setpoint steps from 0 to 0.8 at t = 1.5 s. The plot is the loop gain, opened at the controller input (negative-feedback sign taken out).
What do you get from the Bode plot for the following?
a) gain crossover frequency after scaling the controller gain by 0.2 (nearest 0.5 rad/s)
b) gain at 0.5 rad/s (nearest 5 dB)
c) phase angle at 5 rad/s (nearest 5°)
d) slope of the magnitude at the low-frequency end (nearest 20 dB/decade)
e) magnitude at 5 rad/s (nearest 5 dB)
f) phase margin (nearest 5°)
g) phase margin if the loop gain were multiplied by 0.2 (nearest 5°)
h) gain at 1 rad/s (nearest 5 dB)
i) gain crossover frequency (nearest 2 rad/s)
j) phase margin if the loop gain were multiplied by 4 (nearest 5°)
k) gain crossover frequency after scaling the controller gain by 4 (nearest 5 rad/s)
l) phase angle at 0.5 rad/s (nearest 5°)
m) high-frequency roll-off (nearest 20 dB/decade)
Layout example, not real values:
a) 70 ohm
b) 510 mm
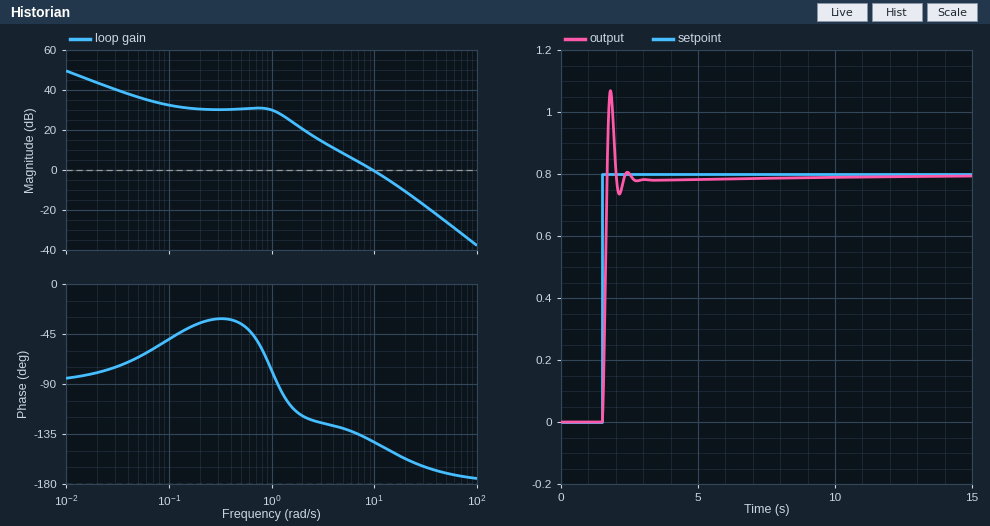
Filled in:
a) 3.0 rad/s
b) 30 dB
c) -130°
d) -20 dB/decade
e) 10 dB
f) 40°
g) 55°
h) 30 dB
i) 10 rad/s
j) 20°
k) 20 rad/s
l) -35°
m) -40 dB/decade
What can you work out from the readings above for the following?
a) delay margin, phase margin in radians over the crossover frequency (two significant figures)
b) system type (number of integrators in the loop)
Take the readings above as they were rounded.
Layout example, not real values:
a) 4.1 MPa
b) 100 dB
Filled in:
a) 0.070 s
b) 1
